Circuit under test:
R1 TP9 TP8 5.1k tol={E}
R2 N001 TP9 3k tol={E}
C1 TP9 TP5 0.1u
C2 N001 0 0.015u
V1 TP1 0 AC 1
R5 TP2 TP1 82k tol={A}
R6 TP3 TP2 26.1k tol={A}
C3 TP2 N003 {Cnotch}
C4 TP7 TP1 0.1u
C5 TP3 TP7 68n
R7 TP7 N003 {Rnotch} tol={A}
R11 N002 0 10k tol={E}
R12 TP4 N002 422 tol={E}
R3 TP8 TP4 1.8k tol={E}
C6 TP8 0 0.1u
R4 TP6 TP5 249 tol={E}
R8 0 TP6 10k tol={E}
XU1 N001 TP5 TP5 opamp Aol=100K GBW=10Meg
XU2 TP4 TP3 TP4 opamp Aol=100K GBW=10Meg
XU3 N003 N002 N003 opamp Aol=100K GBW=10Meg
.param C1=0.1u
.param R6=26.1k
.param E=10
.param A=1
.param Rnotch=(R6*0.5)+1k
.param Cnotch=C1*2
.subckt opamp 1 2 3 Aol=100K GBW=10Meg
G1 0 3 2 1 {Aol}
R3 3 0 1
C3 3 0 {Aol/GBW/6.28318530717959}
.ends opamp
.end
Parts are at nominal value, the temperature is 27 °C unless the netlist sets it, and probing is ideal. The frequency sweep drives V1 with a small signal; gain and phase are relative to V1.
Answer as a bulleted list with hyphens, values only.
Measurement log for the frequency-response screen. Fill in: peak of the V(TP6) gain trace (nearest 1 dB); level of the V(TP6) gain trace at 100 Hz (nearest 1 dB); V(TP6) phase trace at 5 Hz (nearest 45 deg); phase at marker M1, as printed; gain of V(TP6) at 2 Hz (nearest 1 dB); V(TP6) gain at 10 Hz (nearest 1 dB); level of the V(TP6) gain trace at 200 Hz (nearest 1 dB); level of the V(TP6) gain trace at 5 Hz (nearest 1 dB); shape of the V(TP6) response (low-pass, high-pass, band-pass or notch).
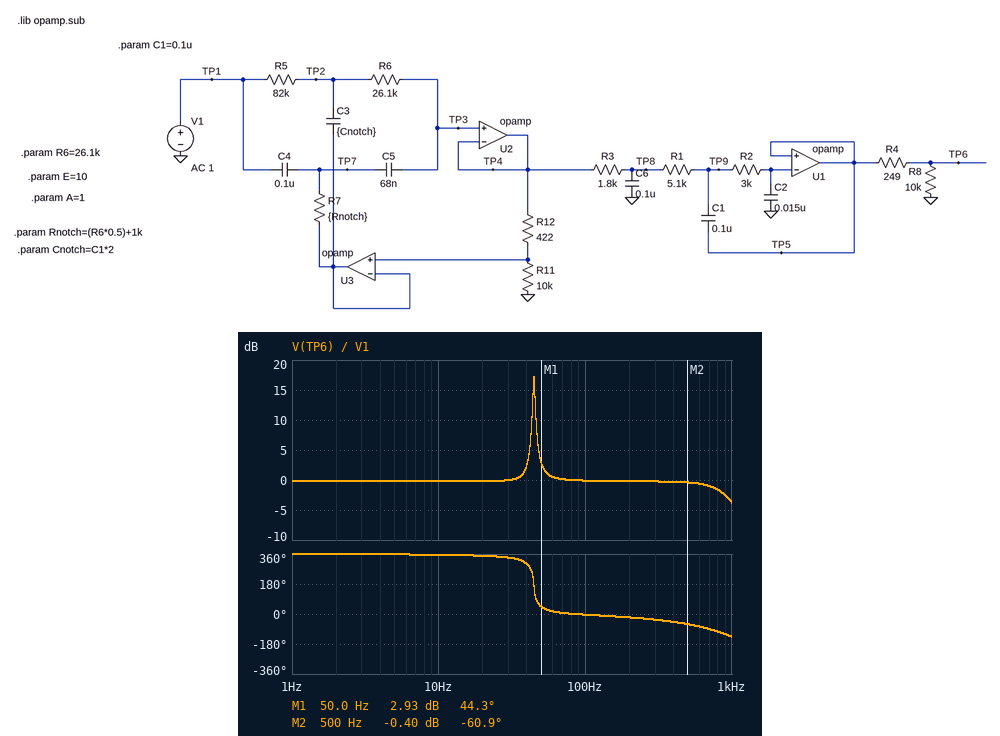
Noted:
- 17 dB
- 0 dB
- 360 deg
- 44.3 deg
- 0 dB
- 0 dB
- 0 dB
- 0 dB
- band-pass
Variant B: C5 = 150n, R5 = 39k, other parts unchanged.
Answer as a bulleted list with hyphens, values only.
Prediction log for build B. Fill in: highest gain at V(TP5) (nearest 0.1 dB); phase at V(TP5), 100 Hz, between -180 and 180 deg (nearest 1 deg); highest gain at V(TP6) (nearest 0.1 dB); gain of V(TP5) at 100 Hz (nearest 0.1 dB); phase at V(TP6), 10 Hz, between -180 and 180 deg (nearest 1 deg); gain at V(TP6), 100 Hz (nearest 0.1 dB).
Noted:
- 0 dB
- -6 deg
- -0.2 dB
- -0.1 dB
- -4 deg
- -0.3 dB
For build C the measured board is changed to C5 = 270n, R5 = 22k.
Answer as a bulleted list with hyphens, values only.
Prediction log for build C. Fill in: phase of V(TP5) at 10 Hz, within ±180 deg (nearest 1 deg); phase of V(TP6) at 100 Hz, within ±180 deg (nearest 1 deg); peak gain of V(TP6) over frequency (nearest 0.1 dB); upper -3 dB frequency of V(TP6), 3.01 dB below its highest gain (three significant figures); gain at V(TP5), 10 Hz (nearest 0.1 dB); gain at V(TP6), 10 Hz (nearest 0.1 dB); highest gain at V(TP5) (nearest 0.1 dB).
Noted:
- -4 deg
- -6 deg
- -0.2 dB
- 958 Hz
- -0.1 dB
- -0.3 dB
- 0 dB
